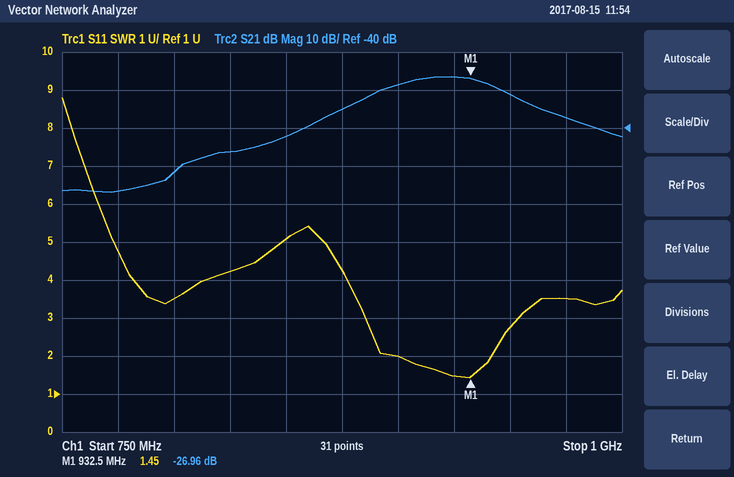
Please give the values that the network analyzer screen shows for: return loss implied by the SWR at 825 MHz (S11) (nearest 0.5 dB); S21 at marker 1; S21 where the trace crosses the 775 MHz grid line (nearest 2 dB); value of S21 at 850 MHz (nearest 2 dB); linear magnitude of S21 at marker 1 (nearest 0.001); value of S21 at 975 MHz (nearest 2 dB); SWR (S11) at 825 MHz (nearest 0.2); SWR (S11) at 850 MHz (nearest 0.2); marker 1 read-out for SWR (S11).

4.0 dB
-26.96 dB
-56 dB
-42 dB
0.045
-38 dB
4.2
5.0
1.45
